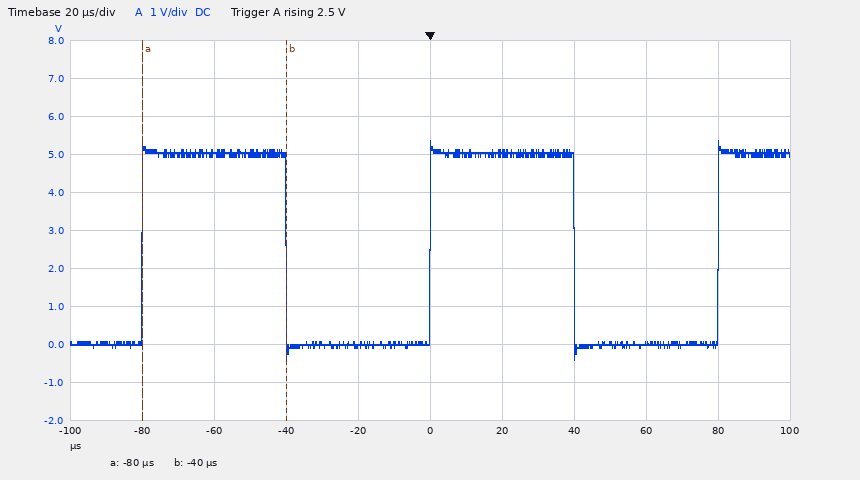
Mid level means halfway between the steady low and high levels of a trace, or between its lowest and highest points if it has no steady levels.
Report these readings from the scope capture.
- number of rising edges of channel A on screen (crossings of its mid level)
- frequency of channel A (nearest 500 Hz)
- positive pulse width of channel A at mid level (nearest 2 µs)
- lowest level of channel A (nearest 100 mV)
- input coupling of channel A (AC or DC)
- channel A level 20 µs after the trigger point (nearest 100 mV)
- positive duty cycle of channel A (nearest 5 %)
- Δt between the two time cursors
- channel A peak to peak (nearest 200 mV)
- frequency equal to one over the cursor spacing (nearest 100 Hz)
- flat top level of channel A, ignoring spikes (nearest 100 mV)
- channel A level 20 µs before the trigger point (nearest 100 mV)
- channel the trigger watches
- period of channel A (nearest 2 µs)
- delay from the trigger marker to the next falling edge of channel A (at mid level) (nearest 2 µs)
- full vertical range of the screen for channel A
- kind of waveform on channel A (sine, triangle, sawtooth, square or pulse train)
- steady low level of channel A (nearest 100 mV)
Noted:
3
12.5 kHz
40 µs
-400 mV
DC
5.0 V
50 %
40 µs
5.8 V
25.0 kHz
5.0 V
0.0 V
channel A
80 µs
40 µs
10 V
square
0.0 V
